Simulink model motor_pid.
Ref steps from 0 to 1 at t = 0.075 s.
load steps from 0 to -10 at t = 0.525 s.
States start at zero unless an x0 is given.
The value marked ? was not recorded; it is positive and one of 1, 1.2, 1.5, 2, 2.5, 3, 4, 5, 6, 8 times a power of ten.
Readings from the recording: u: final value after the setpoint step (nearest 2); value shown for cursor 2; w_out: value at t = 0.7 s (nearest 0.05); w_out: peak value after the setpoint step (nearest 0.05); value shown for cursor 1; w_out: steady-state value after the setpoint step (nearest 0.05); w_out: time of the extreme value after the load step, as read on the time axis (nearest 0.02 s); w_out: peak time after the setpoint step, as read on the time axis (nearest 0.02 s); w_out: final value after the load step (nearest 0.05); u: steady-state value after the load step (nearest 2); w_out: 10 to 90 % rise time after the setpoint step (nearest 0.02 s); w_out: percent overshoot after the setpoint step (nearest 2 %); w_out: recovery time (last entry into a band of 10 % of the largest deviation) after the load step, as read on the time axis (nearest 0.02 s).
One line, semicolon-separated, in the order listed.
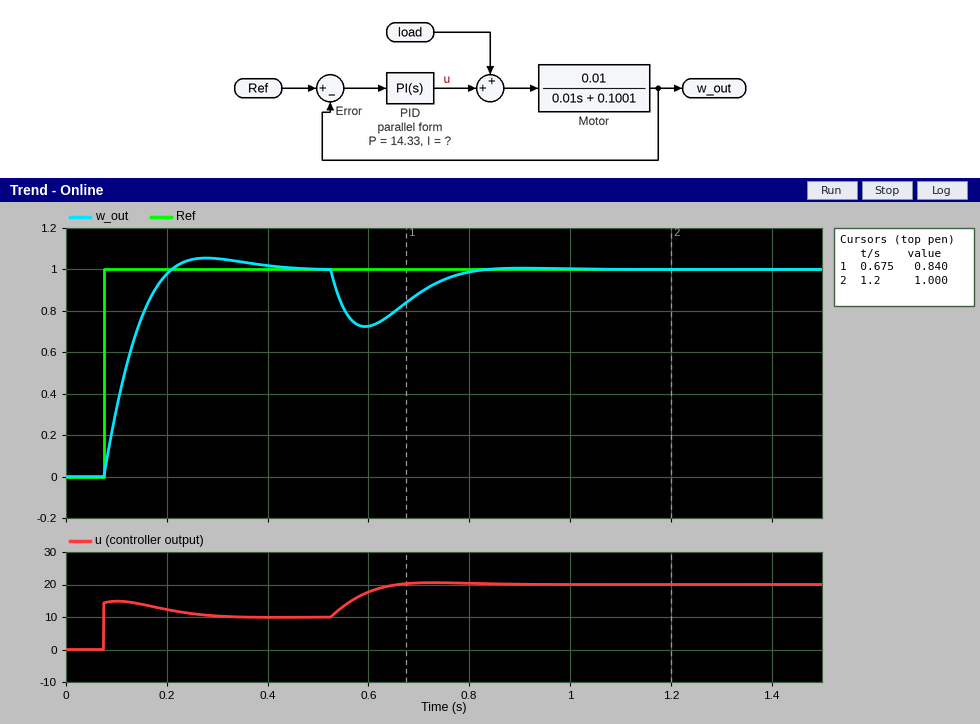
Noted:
10; 1.000; 0.90; 1.05; 0.840; 1.00; 0.60 s; 0.28 s; 1.00; 20; 0.10 s; 6 %; 0.78 s
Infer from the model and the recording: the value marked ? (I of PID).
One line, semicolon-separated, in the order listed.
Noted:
250
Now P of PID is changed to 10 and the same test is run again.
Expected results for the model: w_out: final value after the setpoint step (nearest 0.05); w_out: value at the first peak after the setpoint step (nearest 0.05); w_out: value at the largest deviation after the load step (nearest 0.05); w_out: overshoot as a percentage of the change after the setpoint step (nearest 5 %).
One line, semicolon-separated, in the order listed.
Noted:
1.00; 1.10; 0.70; 10 %
